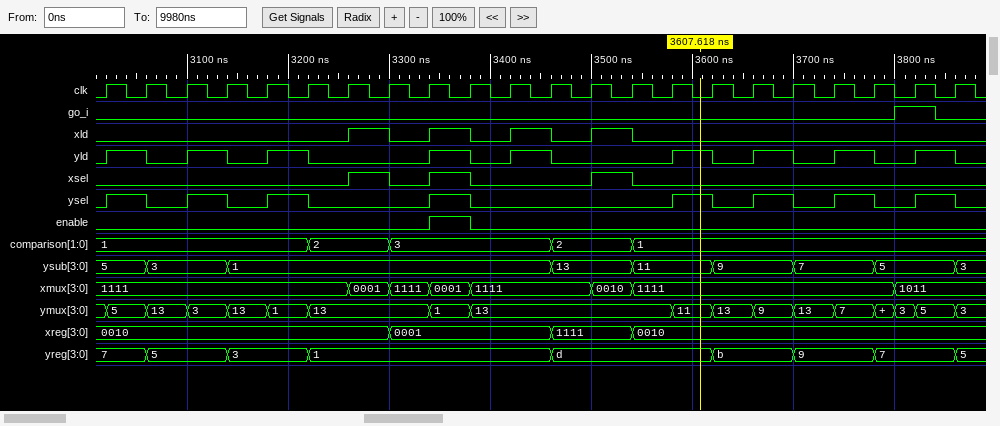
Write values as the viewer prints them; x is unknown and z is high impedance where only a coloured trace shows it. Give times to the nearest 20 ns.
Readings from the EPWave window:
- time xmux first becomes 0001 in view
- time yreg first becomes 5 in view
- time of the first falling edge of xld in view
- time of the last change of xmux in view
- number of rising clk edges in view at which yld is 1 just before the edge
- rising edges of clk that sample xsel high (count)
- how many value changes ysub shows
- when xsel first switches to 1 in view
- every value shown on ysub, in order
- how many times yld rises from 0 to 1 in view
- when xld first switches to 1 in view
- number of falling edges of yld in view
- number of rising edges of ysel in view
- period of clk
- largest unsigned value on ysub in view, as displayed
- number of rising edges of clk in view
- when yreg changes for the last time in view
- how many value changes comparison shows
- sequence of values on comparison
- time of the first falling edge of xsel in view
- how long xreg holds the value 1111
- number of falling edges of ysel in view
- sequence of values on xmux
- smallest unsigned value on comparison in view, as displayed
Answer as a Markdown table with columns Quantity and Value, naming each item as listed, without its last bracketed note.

| Quantity | Value |
|---|---|
| time xmux first becomes 0001 in view | 3260 ns |
| time yreg first becomes 5 in view | 3060 ns |
| time of the first falling edge of xld in view | 3300 ns |
| time of the last change of xmux in view | 3800 ns |
| number of rising clk edges in view at which yld is 1 just before the edge | 9 |
| rising edges of clk that sample xsel high | 3 |
| how many value changes ysub shows | 8 |
| when xsel first switches to 1 in view | 3260 ns |
| every value shown on ysub, in order | 5, 3, 1, 13, 11, 9, 7, 5, 3 |
| how many times yld rises from 0 to 1 in view | 9 |
| when xld first switches to 1 in view | 3260 ns |
| number of falling edges of yld in view | 9 |
| number of rising edges of ysel in view | 8 |
| period of clk | 40 ns |
| largest unsigned value on ysub in view, as displayed | 13 |
| number of rising edges of clk in view | 22 |
| when yreg changes for the last time in view | 3860 ns |
| how many value changes comparison shows | 4 |
| sequence of values on comparison | 1, 2, 3, 2, 1 |
| time of the first falling edge of xsel in view | 3300 ns |
| how long xreg holds the value 1111 | 80 ns |
| number of falling edges of ysel in view | 8 |
| sequence of values on xmux | 1111, 0001, 1111, 0001, 1111, 0010, 1111, 1011 |
| smallest unsigned value on comparison in view, as displayed | 1 |
